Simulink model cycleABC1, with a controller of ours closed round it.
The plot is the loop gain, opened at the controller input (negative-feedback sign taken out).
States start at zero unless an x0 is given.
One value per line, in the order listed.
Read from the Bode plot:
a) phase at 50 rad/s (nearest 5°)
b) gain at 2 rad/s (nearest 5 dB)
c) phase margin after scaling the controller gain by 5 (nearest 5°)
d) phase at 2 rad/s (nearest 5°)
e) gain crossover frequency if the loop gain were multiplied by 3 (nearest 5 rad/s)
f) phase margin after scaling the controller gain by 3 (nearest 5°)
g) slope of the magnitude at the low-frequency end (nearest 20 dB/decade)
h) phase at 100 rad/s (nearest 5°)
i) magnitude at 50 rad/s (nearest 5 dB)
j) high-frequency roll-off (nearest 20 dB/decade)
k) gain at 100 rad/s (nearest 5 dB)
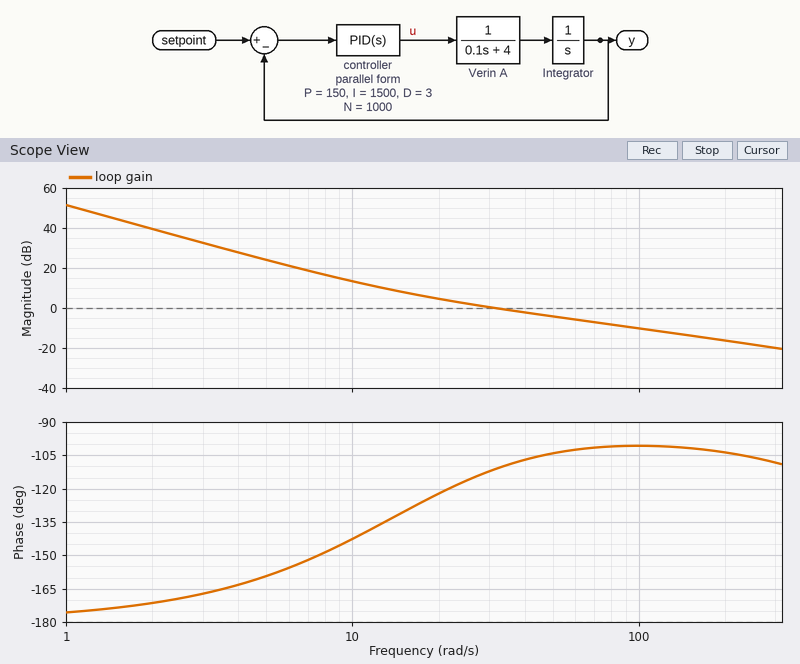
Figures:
-105°
40 dB
80°
-170°
95 rad/s
80°
-40 dB/decade
-100°
-5 dB
-20 dB/decade
-10 dB
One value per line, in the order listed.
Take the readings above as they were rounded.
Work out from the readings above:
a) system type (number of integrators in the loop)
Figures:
2
